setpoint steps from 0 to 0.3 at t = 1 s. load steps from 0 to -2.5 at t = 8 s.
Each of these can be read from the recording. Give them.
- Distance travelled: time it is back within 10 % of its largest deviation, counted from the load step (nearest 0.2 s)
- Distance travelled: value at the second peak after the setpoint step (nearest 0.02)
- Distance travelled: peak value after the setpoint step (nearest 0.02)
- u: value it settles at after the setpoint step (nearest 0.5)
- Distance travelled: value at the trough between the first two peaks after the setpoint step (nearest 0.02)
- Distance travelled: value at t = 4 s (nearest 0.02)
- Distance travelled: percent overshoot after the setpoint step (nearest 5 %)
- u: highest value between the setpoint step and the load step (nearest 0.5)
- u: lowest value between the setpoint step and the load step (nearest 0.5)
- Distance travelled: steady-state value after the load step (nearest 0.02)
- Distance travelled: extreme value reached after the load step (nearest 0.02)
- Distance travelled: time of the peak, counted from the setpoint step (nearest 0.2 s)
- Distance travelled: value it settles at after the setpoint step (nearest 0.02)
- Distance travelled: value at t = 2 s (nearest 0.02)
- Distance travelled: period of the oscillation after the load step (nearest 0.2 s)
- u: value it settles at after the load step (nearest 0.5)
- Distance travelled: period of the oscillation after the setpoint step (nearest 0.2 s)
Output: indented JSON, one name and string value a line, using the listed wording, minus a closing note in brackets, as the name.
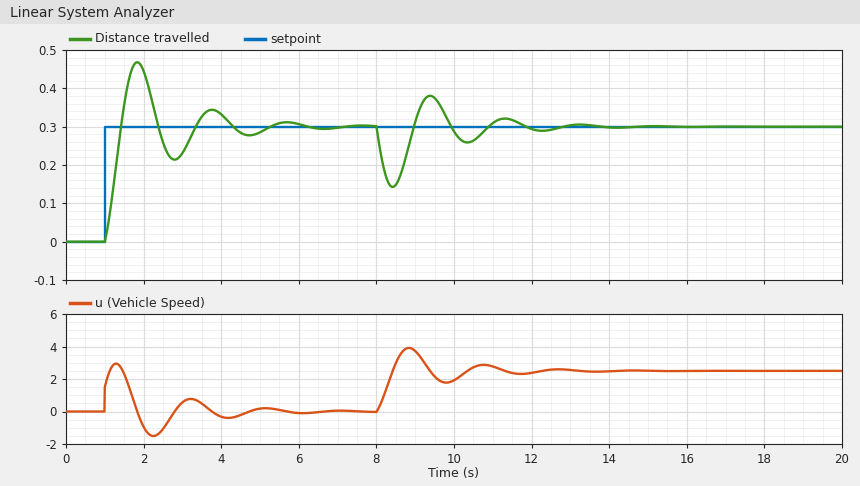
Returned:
{
  "Distance travelled: time it is back within 10 % of its largest deviation, counted from the load step": "3.6 s",
  "Distance travelled: value at the second peak after the setpoint step": "0.34",
  "Distance travelled: peak value after the setpoint step": "0.46",
  "u: value it settles at after the setpoint step": "0.0",
  "Distance travelled: value at the trough between the first two peaks after the setpoint step": "0.22",
  "Distance travelled: value at t = 4 s": "0.34",
  "Distance travelled: percent overshoot after the setpoint step": "55 %",
  "u: highest value between the setpoint step and the load step": "3.0",
  "u: lowest value between the setpoint step and the load step": "-1.5",
  "Distance travelled: steady-state value after the load step": "0.30",
  "Distance travelled: extreme value reached after the load step": "0.14",
  "Distance travelled: time of the peak, counted from the setpoint step": "0.8 s",
  "Distance travelled: value it settles at after the setpoint step": "0.30",
  "Distance travelled: value at t = 2 s": "0.44",
  "Distance travelled: period of the oscillation after the load step": "2.0 s",
  "u: value it settles at after the load step": "2.5",
  "Distance travelled: period of the oscillation after the setpoint step": "2.0 s"
}
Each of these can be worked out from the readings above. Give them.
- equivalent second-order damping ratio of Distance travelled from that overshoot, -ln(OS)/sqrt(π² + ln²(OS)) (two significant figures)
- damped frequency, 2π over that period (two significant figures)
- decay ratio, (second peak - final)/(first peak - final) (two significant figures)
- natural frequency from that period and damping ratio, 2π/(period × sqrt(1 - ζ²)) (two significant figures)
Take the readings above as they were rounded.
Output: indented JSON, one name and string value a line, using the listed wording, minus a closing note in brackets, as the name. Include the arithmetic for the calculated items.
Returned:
{
  "equivalent second-order damping ratio of Distance travelled from that overshoot, -ln(OS)/sqrt(π² + ln²(OS))": "ln(0.55) = -0.598; 0.598 / sqrt(9.870 + 0.357) = 0.19",
  "damped frequency, 2π over that period": "2π / 2 = 3.1 rad/s",
  "decay ratio, (second peak - final)/(first peak - final)": "(0.34 - 0.3) / (0.46 - 0.3) = 0.25",
  "natural frequency from that period and damping ratio, 2π/(period × sqrt(1 - ζ²))": "2π / (2 × sqrt(1 - 0.19²)) = 3.2 rad/s"
}
